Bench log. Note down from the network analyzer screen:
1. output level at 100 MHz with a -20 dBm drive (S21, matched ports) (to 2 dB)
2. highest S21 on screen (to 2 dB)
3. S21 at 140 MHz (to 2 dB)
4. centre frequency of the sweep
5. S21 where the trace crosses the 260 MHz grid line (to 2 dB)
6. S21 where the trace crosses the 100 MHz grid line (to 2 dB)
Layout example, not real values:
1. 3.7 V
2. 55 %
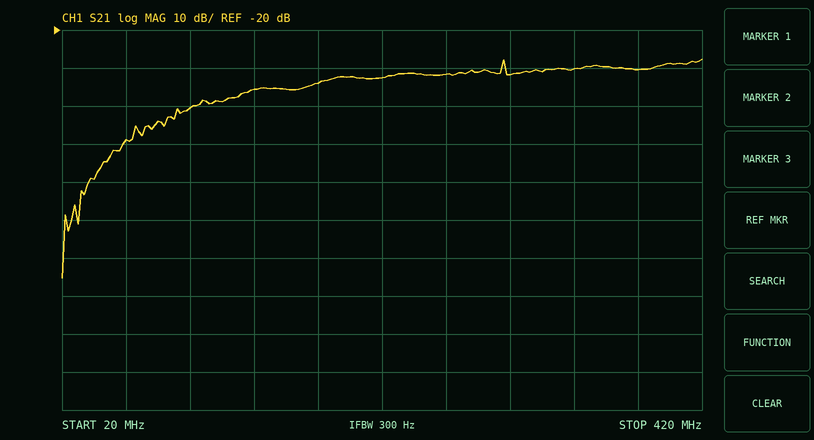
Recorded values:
1. -60 dBm
2. -28 dB
3. -36 dB
4. 220 MHz
5. -32 dB
6. -40 dB
